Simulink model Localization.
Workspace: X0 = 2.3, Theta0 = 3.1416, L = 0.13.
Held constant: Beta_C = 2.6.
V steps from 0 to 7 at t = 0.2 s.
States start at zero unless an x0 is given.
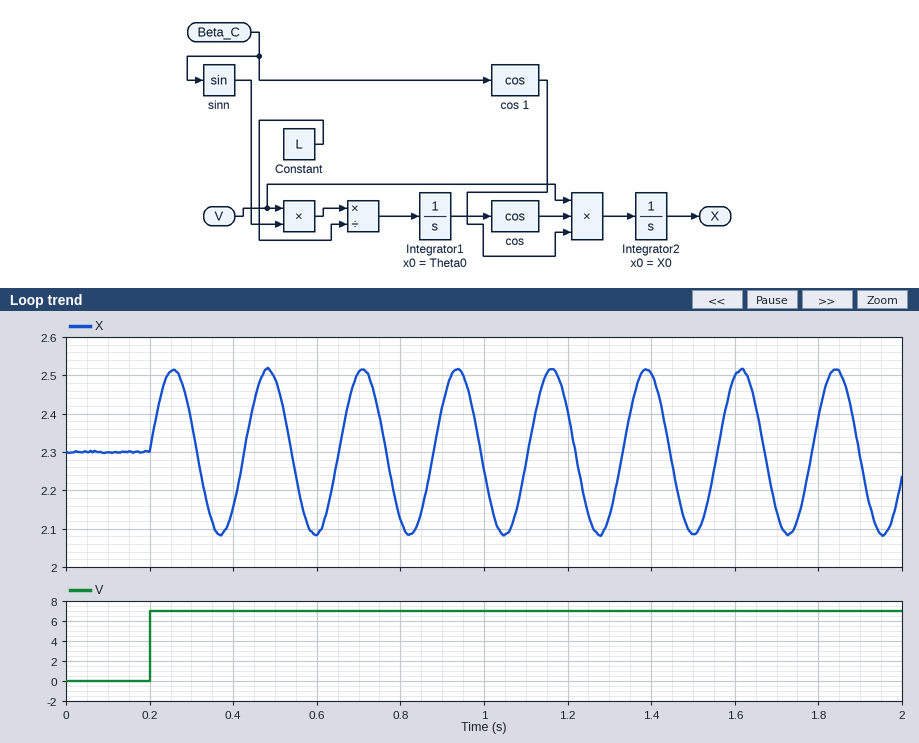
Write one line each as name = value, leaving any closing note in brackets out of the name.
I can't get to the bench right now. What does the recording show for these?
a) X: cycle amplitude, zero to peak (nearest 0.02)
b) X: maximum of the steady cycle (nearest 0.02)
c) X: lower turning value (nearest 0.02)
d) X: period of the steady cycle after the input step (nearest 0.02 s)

X: cycle amplitude, zero to peak = 0.22
X: maximum of the steady cycle = 2.52
X: lower turning value = 2.08
X: period of the steady cycle after the input step = 0.22 s
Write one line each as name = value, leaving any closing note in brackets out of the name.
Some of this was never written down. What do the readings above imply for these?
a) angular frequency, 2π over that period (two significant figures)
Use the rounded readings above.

angular frequency, 2π over that period = 29 rad/s
